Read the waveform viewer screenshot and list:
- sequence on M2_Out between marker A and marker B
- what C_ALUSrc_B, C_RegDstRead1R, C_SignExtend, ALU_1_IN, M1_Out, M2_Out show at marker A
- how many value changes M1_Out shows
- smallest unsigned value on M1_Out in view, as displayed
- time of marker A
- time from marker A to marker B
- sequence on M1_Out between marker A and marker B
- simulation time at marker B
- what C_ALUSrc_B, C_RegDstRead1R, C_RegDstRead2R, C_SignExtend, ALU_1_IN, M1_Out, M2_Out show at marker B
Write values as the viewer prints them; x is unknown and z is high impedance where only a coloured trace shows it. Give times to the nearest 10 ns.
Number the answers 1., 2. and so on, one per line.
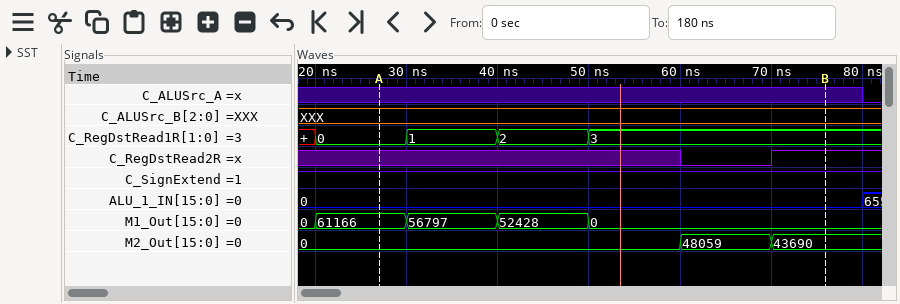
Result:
1. 0, 48059, 43690
2. C_ALUSrc_B=XXX, C_RegDstRead1R=0, C_SignExtend=1, ALU_1_IN=0, M1_Out=61166, M2_Out=0
3. 4
4. 0
5. 30 ns
6. 50 ns
7. 61166, 56797, 52428, 0
8. 80 ns
9. C_ALUSrc_B=XXX, C_RegDstRead1R=3, C_RegDstRead2R=1, C_SignExtend=1, ALU_1_IN=0, M1_Out=0, M2_Out=43690
